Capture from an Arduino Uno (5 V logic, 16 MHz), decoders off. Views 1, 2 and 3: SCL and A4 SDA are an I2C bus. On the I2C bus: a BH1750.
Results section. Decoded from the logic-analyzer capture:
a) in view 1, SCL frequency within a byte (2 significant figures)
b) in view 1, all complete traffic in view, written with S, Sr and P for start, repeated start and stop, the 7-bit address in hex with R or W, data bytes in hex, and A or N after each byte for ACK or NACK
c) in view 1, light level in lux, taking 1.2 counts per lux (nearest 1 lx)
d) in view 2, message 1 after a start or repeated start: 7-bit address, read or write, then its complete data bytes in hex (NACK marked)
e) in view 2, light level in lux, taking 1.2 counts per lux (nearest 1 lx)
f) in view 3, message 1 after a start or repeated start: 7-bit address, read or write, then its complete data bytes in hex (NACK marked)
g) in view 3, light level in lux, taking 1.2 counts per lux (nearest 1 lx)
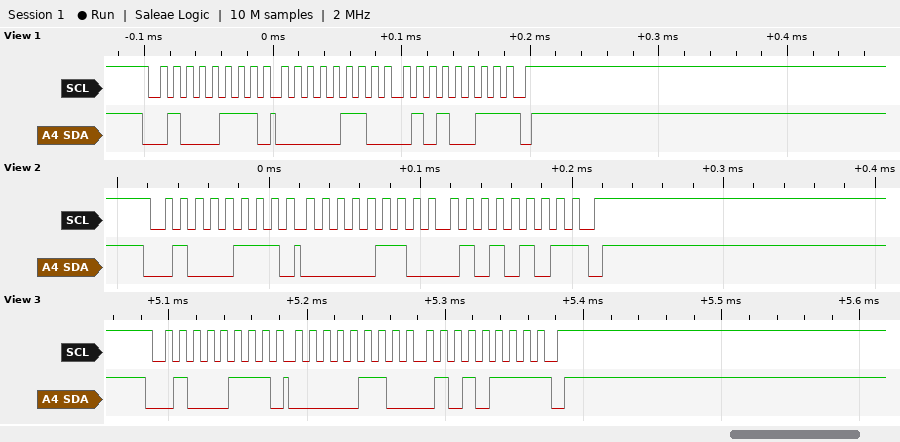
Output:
100 kHz
S 23R A 06 A 53 N P
1349 lx
0x23 read: 06 55 NACK
1351 lx
0x23 read: 06 57 NACK
1352 lx
